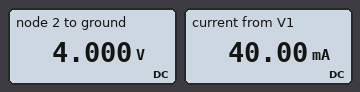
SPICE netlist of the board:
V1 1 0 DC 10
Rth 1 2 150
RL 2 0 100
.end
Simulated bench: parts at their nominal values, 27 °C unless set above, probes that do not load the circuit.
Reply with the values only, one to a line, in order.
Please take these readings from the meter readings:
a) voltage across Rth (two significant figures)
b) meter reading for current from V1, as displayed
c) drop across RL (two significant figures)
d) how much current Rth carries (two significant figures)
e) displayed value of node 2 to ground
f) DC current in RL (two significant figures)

6.0 V
40.00 mA
4.0 V
40 mA
4.000 V
40 mA
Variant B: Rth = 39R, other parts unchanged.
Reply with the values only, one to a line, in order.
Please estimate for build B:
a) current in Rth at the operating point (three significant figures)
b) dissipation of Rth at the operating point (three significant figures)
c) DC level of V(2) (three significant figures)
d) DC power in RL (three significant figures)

71.9 mA
202 mW
7.19 V
518 mW
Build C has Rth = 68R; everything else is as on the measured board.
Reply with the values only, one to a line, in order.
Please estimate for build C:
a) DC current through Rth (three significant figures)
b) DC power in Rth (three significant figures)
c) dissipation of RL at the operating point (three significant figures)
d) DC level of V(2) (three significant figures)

59.5 mA
241 mW
354 mW
5.95 V
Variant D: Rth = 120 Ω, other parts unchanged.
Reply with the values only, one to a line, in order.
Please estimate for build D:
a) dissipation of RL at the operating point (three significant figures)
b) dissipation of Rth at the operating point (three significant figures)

207 mW
248 mW
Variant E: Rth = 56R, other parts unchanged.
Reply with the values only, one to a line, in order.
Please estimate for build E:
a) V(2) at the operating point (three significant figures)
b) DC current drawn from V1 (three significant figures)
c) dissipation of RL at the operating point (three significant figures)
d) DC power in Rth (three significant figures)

6.41 V
64.1 mA
411 mW
230 mW
